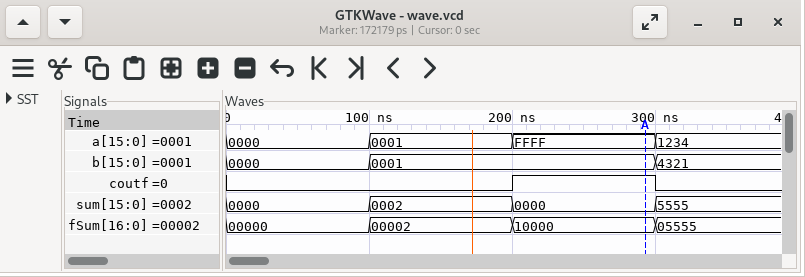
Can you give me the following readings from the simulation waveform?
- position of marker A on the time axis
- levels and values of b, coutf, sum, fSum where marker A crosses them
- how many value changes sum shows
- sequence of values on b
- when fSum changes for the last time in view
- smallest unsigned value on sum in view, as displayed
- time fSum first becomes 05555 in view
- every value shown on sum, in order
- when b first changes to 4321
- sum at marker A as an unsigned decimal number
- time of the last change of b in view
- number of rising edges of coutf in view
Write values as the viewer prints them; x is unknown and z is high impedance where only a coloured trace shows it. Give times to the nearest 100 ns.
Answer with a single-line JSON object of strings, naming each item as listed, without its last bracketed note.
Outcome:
{"position of marker A on the time axis": "300 ns", "levels and values of b, coutf, sum, fSum where marker A crosses them": "b=0001, coutf=1, sum=0000, fSum=10000", "how many value changes sum shows": "3", "sequence of values on b": "0000, 0001, 4321", "when fSum changes for the last time in view": "300 ns", "smallest unsigned value on sum in view, as displayed": "0000", "time fSum first becomes 05555 in view": "300 ns", "every value shown on sum, in order": "0000, 0002, 0000, 5555", "when b first changes to 4321": "300 ns", "sum at marker A as an unsigned decimal number": "0", "time of the last change of b in view": "300 ns", "number of rising edges of coutf in view": "1"}
